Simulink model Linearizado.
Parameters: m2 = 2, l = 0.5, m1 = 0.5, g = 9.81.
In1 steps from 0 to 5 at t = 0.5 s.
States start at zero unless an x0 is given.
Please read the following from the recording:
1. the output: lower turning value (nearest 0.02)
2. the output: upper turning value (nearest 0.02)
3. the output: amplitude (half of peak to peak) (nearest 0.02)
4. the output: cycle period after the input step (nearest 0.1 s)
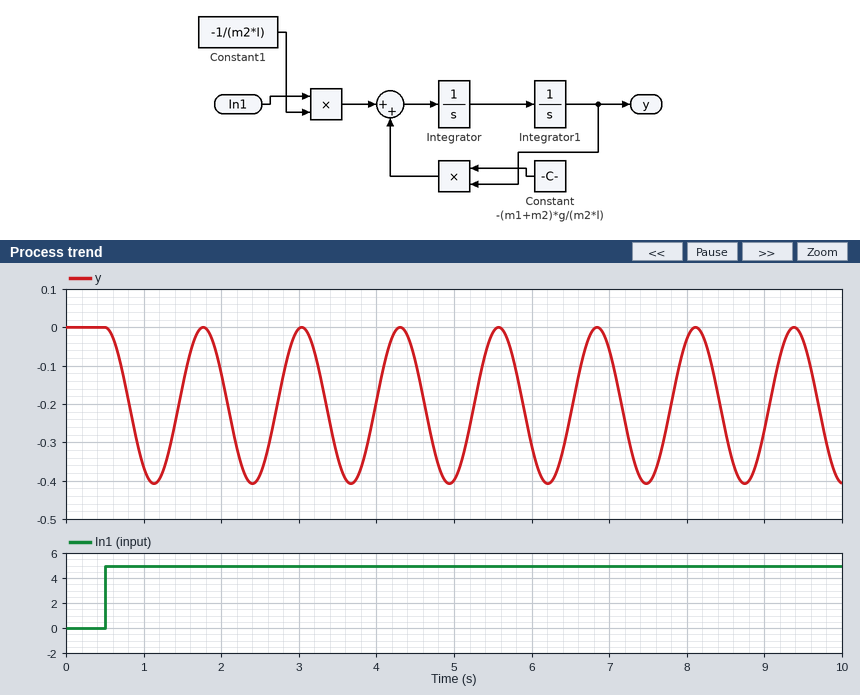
-0.40
0.00
0.20
1.3 s
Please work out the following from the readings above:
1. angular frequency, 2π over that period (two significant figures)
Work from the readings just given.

4.8 rad/s
